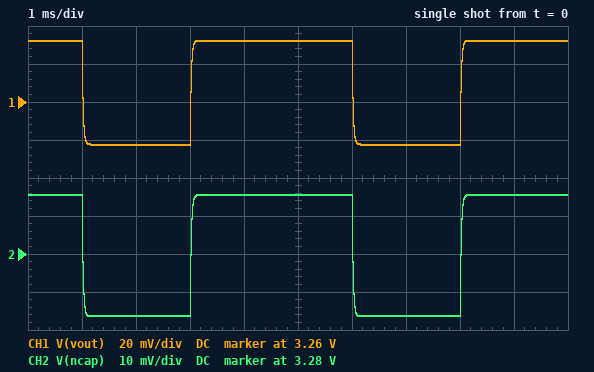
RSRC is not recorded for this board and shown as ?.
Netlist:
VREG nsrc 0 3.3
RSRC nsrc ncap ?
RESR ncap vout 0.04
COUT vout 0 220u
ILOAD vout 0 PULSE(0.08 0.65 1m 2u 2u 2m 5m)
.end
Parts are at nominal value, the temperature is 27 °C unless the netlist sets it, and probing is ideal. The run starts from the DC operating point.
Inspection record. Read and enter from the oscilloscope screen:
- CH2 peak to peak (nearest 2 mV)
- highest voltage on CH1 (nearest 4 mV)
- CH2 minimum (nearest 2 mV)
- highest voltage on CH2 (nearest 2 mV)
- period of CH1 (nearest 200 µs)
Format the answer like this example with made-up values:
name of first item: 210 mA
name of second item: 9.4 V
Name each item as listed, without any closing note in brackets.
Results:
CH2 peak to peak: 32 mV
highest voltage on CH1: 3.292 V
CH2 minimum: 3.264 V
highest voltage on CH2: 3.296 V
period of CH1: 5.0 ms
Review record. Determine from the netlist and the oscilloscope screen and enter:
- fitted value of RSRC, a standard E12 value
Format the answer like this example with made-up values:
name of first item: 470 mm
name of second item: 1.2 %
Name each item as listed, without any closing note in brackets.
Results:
fitted value of RSRC, a standard E12 value: 0.056 Ω
